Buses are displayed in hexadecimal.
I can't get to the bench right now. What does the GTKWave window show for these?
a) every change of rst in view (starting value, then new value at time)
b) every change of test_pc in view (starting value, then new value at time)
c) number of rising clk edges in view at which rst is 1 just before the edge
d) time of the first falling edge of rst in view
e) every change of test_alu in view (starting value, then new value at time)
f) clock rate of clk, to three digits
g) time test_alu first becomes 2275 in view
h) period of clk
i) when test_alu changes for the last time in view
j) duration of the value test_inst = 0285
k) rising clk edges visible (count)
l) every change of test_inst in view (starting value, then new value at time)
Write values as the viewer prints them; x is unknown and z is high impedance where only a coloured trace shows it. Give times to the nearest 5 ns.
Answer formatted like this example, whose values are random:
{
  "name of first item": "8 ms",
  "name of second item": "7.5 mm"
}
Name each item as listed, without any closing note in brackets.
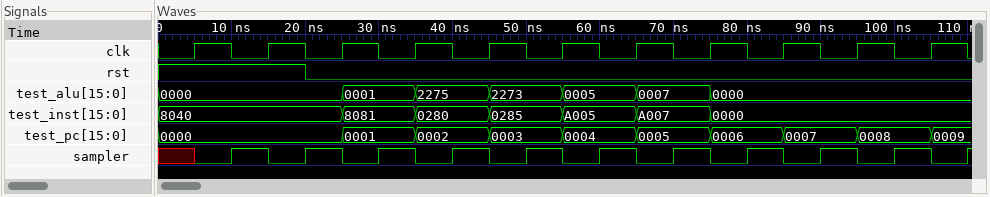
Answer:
{
  "every change of rst in view": "1, 0 at 20 ns",
  "every change of test_pc in view": "0000, 0001 at 25 ns, 0002 at 35 ns, 0003 at 45 ns, 0004 at 55 ns, 0005 at 65 ns, 0006 at 75 ns, 0007 at 85 ns, 0008 at 95 ns, 0009 at 105 ns",
  "number of rising clk edges in view at which rst is 1 just before the edge": "2",
  "time of the first falling edge of rst in view": "20 ns",
  "every change of test_alu in view": "0000, 0001 at 25 ns, 2275 at 35 ns, 2273 at 45 ns, 0005 at 55 ns, 0007 at 65 ns, 0000 at 75 ns",
  "clock rate of clk, to three digits": "100 MHz",
  "time test_alu first becomes 2275 in view": "35 ns",
  "period of clk": "10 ns",
  "when test_alu changes for the last time in view": "75 ns",
  "duration of the value test_inst = 0285": "10 ns",
  "rising clk edges visible": "11",
  "every change of test_inst in view": "8040, 8081 at 25 ns, 0280 at 35 ns, 0285 at 45 ns, A005 at 55 ns, A007 at 65 ns, 0000 at 75 ns"
}
